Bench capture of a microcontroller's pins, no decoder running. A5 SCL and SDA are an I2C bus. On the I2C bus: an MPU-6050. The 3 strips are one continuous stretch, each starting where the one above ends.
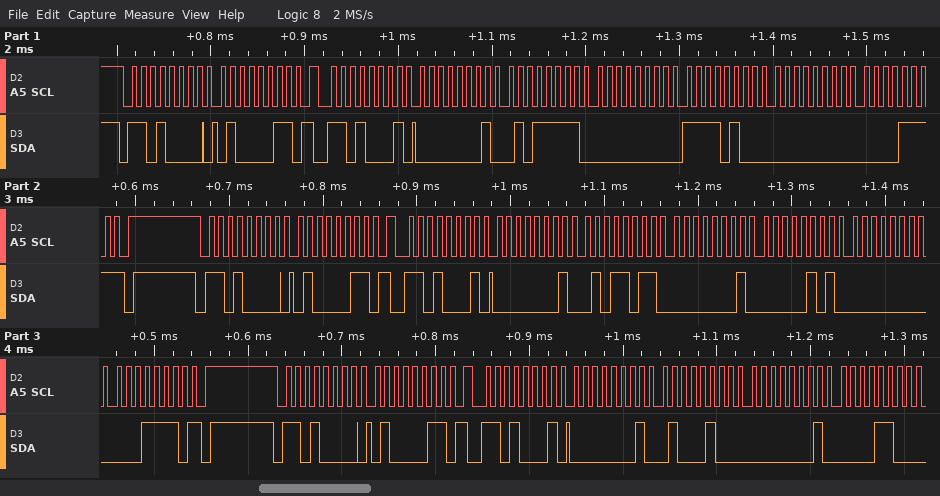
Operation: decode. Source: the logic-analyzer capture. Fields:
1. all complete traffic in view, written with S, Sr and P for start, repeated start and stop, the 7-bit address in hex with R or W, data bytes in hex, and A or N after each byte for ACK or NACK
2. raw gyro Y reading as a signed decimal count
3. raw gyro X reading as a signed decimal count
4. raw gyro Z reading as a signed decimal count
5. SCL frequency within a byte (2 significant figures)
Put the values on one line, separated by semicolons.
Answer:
S 68W A 43 A Sr 68R A 01 A 5F A 00 A F4 A 00 A 0F N P S 68W A 43 A Sr 68R A 01 A 5B A 01 A 05 A 00 A 1E N P S 68W A 43 A Sr 68R A 01 A 44 A 01 A 0C A; 244; 351; 15; 100 kHz
